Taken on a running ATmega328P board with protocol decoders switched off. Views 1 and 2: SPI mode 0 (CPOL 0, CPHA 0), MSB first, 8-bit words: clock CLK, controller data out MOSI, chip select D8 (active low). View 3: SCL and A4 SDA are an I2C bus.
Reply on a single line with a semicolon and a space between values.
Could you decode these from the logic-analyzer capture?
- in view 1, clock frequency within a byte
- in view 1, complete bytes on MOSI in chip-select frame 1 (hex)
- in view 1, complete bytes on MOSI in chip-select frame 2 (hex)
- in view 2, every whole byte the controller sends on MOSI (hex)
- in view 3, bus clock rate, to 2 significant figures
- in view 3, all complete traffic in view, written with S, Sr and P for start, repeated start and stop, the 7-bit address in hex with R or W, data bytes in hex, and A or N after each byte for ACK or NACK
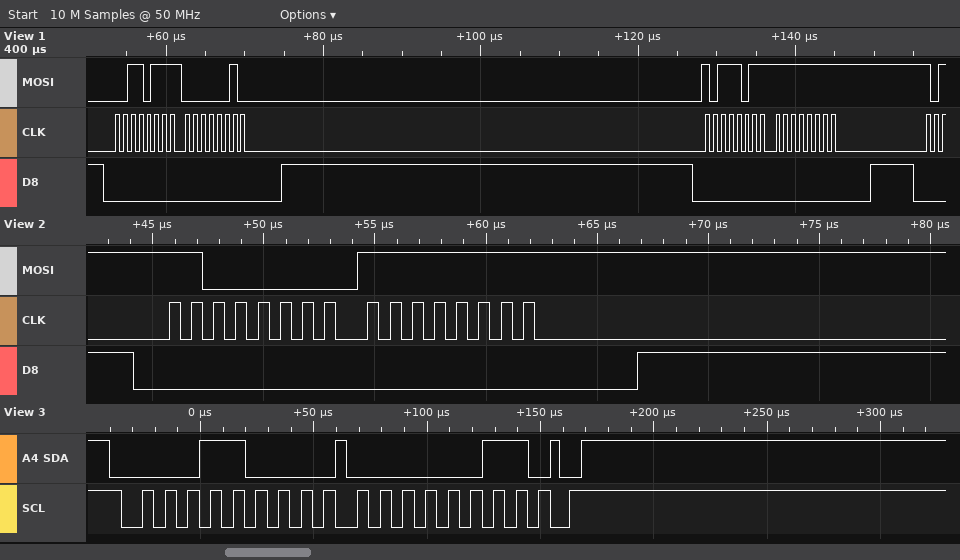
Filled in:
1 MHz; 0x37 0x02; 0xBB 0xFF; C0 FF; 100 kHz; S 0CW A 03 A P
